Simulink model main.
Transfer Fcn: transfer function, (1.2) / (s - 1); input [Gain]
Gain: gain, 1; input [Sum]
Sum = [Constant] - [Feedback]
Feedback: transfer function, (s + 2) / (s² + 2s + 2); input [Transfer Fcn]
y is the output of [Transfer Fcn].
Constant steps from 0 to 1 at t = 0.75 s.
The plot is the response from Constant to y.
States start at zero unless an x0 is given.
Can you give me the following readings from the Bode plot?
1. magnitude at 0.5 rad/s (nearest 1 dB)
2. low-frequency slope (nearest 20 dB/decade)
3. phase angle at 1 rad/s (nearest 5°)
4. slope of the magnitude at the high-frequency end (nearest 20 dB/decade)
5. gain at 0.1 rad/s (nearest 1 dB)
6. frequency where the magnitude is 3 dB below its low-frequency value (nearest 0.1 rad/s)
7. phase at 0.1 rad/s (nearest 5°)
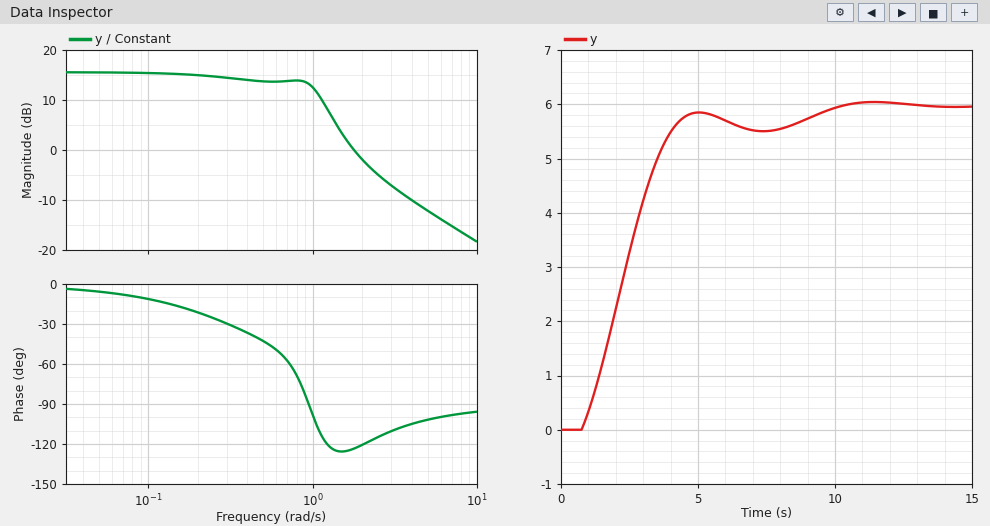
14 dB
0 dB/decade
-100°
-20 dB/decade
15 dB
1.0 rad/s
-10°
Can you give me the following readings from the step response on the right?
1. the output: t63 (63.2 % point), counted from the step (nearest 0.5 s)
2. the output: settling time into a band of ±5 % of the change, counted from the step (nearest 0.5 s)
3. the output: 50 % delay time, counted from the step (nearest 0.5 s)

2.0 s
8.0 s
1.5 s
